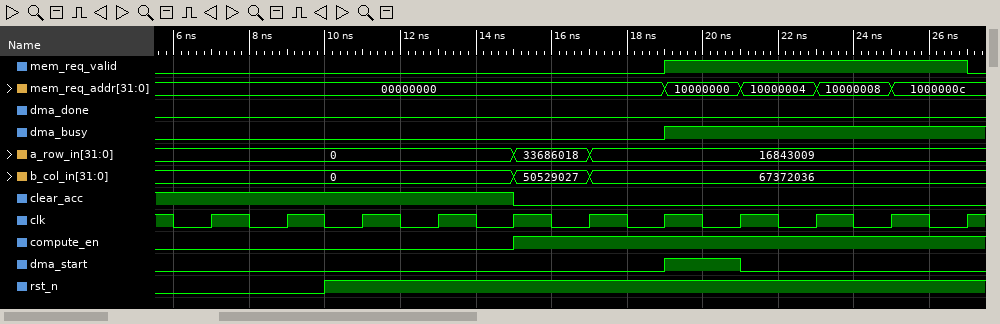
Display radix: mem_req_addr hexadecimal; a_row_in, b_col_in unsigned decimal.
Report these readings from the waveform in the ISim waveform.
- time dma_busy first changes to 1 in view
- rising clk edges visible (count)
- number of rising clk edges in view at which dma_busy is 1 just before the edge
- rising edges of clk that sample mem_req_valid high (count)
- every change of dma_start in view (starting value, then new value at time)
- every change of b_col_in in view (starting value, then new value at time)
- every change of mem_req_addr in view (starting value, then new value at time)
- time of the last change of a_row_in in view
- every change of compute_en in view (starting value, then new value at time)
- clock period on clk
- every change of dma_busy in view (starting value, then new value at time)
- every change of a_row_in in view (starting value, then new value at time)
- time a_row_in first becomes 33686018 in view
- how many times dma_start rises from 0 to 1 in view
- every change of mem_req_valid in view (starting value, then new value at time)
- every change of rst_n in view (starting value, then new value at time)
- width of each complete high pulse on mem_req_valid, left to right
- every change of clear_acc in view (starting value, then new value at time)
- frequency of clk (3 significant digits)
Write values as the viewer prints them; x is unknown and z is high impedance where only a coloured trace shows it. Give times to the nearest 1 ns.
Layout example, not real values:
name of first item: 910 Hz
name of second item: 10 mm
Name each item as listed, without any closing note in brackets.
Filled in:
time dma_busy first changes to 1 in view: 19 ns
rising clk edges visible: 11
number of rising clk edges in view at which dma_busy is 1 just before the edge: 4
rising edges of clk that sample mem_req_valid high: 4
every change of dma_start in view: 0, 1 at 19 ns, 0 at 21 ns
every change of b_col_in in view: 0, 50529027 at 15 ns, 67372036 at 17 ns
every change of mem_req_addr in view: 00000000, 10000000 at 19 ns, 10000004 at 21 ns, 10000008 at 23 ns, 1000000c at 25 ns
time of the last change of a_row_in in view: 17 ns
every change of compute_en in view: 0, 1 at 15 ns
clock period on clk: 2 ns
every change of dma_busy in view: 0, 1 at 19 ns
every change of a_row_in in view: 0, 33686018 at 15 ns, 16843009 at 17 ns
time a_row_in first becomes 33686018 in view: 15 ns
how many times dma_start rises from 0 to 1 in view: 1
every change of mem_req_valid in view: 0, 1 at 19 ns, 0 at 27 ns
every change of rst_n in view: 0, 1 at 10 ns
width of each complete high pulse on mem_req_valid, left to right: 8 ns
every change of clear_acc in view: 1, 0 at 15 ns
frequency of clk: 500 MHz
